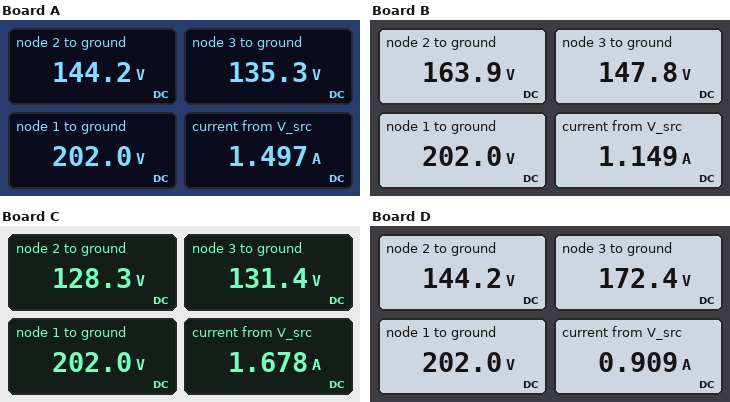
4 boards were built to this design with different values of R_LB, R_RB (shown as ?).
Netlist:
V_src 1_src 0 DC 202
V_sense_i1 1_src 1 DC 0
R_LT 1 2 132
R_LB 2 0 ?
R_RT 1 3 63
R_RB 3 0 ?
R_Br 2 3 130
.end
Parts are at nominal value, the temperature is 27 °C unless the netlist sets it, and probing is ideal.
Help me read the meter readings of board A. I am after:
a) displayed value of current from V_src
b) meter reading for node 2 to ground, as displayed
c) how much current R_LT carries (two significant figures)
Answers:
1.497 A
144.2 V
440 mA
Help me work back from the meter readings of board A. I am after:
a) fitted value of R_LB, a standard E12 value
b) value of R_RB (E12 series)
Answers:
390 Ω
120 Ω
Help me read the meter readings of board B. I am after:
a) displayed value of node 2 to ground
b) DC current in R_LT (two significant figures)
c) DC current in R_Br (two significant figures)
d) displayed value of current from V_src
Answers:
163.9 V
290 mA
120 mA
1.149 A
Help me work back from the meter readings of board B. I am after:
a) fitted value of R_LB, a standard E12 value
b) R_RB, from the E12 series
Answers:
1 kΩ
150 Ω
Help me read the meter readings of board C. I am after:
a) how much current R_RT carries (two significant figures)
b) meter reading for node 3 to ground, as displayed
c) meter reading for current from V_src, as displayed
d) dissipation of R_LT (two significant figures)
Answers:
1.1 A
131.4 V
1.678 A
41 W
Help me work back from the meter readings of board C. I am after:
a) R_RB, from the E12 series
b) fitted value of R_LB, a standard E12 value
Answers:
120 Ω
220 Ω
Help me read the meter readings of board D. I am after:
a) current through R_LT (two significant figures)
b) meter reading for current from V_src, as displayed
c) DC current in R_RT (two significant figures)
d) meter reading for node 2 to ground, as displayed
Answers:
440 mA
0.909 A
470 mA
144.2 V
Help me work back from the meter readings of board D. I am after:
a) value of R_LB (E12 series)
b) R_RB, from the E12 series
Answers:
220 Ω
680 Ω
